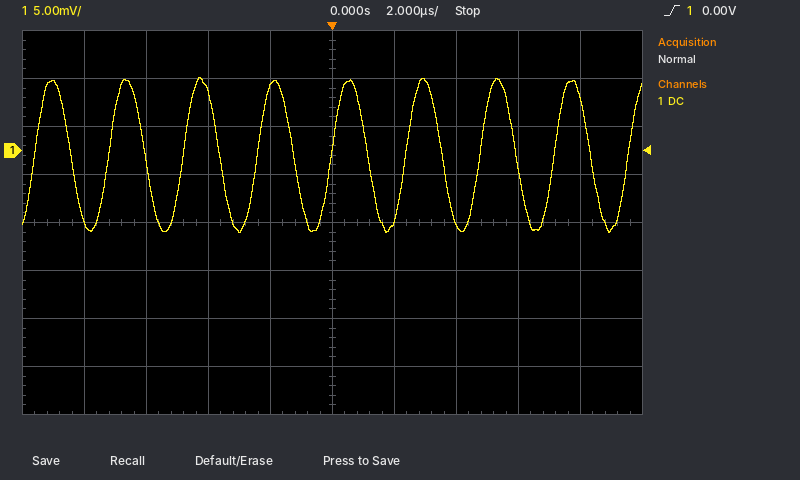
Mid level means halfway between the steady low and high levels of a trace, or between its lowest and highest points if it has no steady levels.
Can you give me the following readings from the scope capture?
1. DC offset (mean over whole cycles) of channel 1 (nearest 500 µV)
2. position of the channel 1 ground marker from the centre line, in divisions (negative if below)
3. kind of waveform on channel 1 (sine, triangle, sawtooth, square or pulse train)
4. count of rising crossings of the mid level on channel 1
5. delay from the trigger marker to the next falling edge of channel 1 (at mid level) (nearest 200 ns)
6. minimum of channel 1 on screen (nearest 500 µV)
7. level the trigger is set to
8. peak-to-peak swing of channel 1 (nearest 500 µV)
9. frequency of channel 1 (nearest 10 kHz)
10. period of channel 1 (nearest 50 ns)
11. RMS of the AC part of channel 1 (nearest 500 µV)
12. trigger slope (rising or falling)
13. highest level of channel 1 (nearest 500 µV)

-500 µV
+1.5 div
sine
9
1.2 µs
-8.5 mV
0.00 V
16.0 mV
420 kHz
2.40 µs
5.5 mV
rising
7.5 mV
